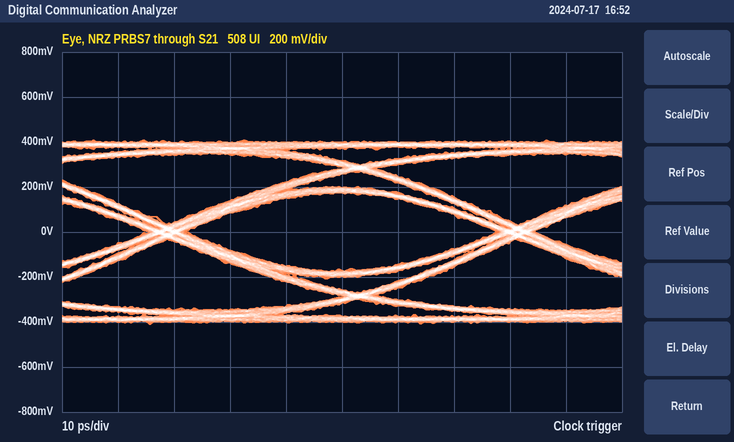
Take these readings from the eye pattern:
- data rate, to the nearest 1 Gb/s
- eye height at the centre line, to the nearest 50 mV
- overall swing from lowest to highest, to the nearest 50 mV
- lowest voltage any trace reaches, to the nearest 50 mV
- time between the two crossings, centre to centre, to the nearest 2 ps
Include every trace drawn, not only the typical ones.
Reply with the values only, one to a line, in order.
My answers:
16 Gb/s
350 mV
800 mV
-400 mV
62 ps
